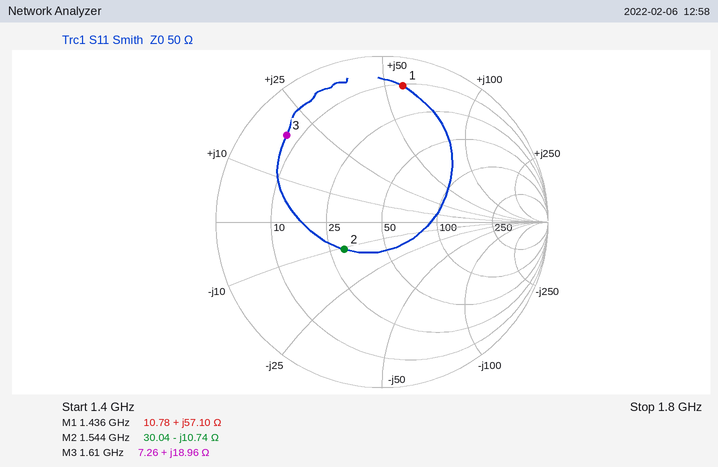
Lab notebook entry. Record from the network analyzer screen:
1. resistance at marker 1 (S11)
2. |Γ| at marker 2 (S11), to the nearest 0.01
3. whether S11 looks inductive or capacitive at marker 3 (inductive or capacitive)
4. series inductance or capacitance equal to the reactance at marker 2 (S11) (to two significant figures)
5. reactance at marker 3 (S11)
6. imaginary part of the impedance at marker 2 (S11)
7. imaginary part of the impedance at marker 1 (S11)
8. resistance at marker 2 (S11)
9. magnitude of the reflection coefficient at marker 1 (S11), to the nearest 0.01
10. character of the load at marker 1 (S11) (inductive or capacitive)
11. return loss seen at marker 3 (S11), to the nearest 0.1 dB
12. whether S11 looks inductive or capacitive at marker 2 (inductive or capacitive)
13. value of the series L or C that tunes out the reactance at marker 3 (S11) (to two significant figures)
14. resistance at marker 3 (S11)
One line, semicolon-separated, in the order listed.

10.78 Ω; 0.28; inductive; 9.6 pF; +18.96 Ω; -10.74 Ω; +57.10 Ω; 30.04 Ω; 0.83; inductive; 2.2 dB; capacitive; 5.2 pF; 7.26 Ω
